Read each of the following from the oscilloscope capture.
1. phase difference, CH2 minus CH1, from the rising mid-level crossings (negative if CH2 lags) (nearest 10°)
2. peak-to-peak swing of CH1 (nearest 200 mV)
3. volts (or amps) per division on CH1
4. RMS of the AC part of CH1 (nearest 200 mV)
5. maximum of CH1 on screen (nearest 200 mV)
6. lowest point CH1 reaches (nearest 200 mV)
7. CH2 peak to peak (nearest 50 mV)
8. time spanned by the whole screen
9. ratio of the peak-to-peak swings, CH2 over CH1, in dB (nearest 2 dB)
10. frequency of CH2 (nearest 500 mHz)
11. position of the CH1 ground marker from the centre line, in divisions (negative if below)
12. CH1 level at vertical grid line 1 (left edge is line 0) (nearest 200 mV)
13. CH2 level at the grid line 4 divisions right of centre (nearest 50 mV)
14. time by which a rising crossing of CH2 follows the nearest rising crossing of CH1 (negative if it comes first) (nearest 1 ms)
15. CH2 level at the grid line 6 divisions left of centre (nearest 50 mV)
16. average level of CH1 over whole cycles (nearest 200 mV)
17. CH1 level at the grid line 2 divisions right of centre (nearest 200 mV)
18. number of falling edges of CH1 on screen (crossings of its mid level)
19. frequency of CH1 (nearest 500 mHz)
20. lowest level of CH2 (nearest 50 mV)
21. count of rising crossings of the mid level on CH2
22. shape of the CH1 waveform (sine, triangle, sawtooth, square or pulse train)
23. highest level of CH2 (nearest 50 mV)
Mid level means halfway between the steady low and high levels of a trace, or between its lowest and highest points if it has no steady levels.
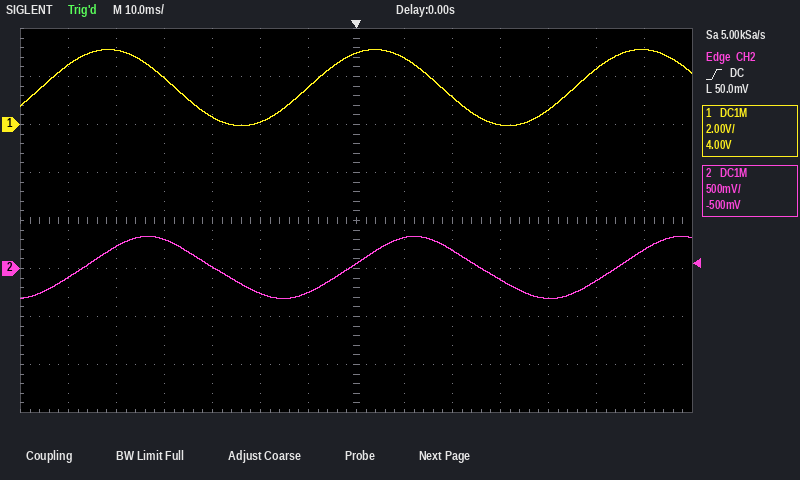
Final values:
-60°
3.2 V
2 V
1.2 V
3.2 V
0.0 V
650 mV
140 ms
-14 dB
18.0 Hz
+2.0 div
2.4 V
-300 mV
+9 ms
-100 mV
1.6 V
1.2 V
2
18.0 Hz
-300 mV
3
sine
350 mV
